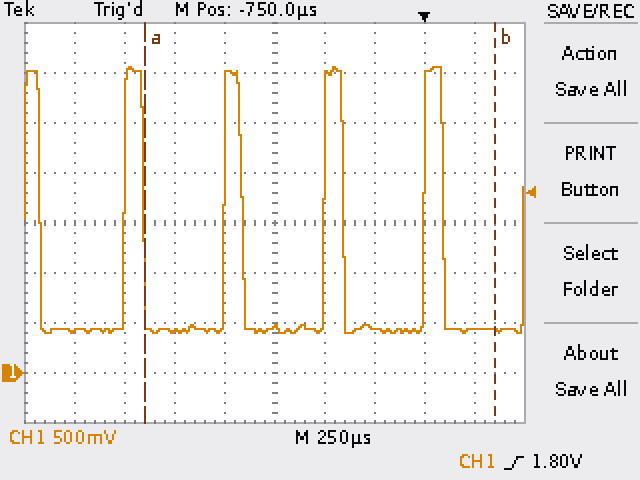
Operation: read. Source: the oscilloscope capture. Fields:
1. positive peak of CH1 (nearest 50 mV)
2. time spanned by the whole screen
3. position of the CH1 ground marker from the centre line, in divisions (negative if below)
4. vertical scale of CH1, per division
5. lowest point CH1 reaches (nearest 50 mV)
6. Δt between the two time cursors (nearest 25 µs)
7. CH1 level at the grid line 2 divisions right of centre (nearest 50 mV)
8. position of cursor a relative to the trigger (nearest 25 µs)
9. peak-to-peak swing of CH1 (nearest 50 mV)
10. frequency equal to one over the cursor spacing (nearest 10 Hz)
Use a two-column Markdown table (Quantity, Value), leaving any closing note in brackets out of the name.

| Quantity | Value |
|---|---|
| positive peak of CH1 | 3.05 V |
| time spanned by the whole screen | 2.5 ms |
| position of the CH1 ground marker from the centre line, in divisions | -3.0 div |
| vertical scale of CH1, per division | 500 mV |
| lowest point CH1 reaches | 400 mV |
| Δt between the two time cursors | 1.750 ms |
| CH1 level at the grid line 2 divisions right of centre | 450 mV |
| position of cursor a relative to the trigger | -1.400 ms |
| peak-to-peak swing of CH1 | 2.65 V |
| frequency equal to one over the cursor spacing | 570 Hz |
